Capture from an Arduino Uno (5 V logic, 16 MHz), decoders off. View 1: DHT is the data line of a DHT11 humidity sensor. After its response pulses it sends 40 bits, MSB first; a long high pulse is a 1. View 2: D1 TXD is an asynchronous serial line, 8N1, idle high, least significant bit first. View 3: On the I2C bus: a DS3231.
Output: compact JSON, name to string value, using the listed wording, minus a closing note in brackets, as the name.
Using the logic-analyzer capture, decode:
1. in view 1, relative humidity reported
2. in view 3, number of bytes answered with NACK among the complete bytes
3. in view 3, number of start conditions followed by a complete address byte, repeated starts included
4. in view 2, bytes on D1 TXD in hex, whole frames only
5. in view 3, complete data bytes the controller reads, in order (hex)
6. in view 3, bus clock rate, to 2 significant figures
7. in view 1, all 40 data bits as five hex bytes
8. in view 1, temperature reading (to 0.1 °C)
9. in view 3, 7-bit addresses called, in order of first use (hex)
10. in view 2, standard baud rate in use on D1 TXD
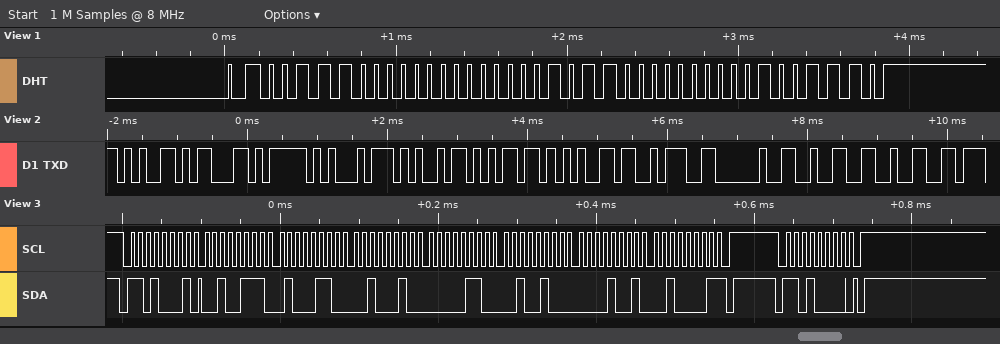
{"in view 1, relative humidity reported": "56 %", "in view 3, number of bytes answered with NACK among the complete bytes": "1", "in view 3, number of start conditions followed by a complete address byte, repeated starts included": "2", "in view 2, bytes on D1 TXD in hex, whole frames only": "65 63 5F 74 69 6D 65 3A 20 32 32", "in view 3, complete data bytes the controller reads, in order": "27 46 22 06 24 09 21", "in view 3, bus clock rate, to 2 significant figures": "100 kHz", "in view 1, all 40 data bits as five hex bytes": "38 00 16 00 4E", "in view 1, temperature reading": "22.0 °C", "in view 3, 7-bit addresses called, in order of first use": "0x68", "in view 2, standard baud rate in use on D1 TXD": "9600 baud"}
